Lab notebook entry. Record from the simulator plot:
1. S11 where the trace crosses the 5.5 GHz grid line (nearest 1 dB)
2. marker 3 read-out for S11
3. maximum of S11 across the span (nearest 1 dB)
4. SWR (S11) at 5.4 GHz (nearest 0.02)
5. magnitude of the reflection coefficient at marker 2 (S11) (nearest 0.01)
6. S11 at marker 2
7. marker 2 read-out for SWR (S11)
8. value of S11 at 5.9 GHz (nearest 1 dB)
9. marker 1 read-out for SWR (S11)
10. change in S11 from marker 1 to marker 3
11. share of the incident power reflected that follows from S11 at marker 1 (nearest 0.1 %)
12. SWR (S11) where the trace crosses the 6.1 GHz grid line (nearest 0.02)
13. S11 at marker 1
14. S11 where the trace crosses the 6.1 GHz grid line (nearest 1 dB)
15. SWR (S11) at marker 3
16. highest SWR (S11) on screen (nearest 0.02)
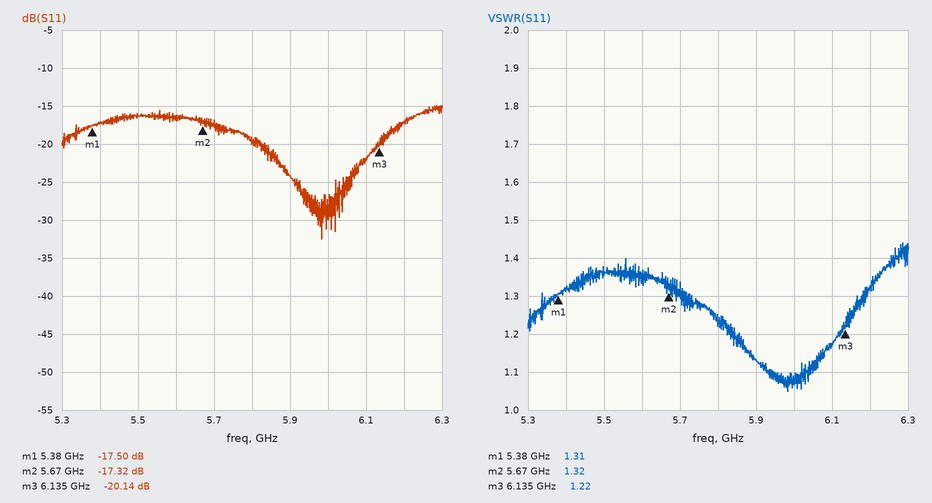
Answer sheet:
-16 dB
-20.14 dB
-15 dB
1.32
0.14
-17.32 dB
1.32
-24 dB
1.31
-2.64 dB
1.8 %
1.18
-17.50 dB
-22 dB
1.22
1.44
